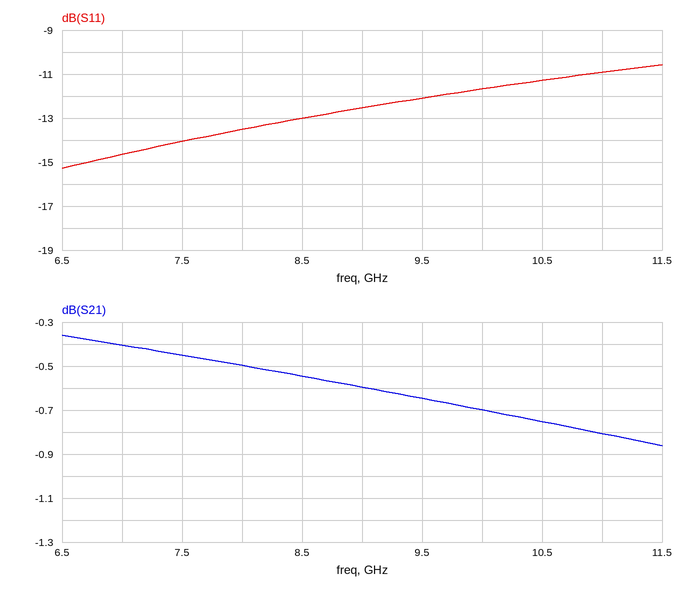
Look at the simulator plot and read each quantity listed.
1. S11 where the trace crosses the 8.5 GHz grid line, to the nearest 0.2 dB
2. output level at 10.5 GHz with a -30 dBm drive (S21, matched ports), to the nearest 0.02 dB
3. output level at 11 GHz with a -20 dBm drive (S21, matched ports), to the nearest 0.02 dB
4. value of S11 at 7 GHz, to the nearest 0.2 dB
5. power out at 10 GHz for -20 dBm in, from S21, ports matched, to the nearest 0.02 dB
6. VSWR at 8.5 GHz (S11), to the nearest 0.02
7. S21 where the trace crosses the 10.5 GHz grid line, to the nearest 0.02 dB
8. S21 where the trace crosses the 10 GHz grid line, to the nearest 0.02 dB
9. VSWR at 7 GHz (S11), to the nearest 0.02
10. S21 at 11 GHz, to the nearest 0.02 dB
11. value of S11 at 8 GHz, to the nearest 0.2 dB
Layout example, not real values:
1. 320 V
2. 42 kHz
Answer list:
1. -13.0 dB
2. -30.76 dBm
3. -20.80 dBm
4. -14.6 dB
5. -20.70 dBm
6. 1.58
7. -0.76 dB
8. -0.70 dB
9. 1.46
10. -0.80 dB
11. -13.6 dB
